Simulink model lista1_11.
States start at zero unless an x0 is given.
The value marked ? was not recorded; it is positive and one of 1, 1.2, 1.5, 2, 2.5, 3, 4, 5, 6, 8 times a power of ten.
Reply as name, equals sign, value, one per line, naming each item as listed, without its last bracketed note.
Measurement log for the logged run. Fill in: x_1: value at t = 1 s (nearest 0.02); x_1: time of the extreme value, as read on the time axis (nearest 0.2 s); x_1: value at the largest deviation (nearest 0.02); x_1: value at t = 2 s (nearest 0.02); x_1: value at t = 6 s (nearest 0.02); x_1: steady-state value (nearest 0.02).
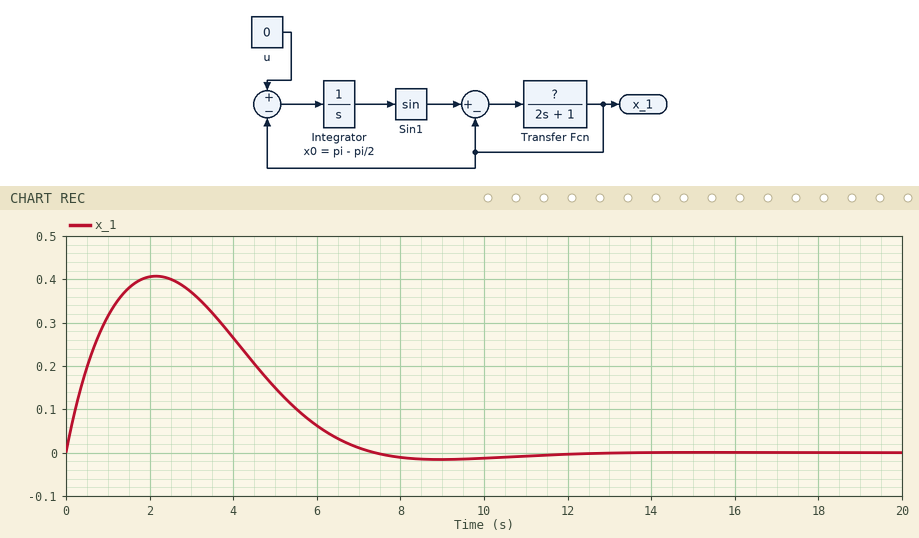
x_1: value at t = 1 s = 0.32
x_1: time of the extreme value, as read on the time axis = 2.2 s
x_1: value at the largest deviation = 0.40
x_1: value at t = 2 s = 0.40
x_1: value at t = 6 s = 0.06
x_1: steady-state value = 0.00
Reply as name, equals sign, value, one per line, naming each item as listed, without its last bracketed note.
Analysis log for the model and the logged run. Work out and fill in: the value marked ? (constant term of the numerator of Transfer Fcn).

the value marked ? = 1
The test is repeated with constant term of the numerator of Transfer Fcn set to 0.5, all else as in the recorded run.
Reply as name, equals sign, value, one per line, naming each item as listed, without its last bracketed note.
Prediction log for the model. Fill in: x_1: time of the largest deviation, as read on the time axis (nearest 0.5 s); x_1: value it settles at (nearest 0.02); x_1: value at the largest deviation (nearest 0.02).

x_1: time of the largest deviation, as read on the time axis = 3.0 s
x_1: value it settles at = 0.00
x_1: value at the largest deviation = 0.28
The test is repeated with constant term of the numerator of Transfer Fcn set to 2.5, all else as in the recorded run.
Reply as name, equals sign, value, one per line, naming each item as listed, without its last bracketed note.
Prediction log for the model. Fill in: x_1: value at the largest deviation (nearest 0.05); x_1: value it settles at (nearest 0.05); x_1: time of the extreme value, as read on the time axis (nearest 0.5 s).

x_1: value at the largest deviation = 0.60
x_1: value it settles at = 0.00
x_1: time of the extreme value, as read on the time axis = 1.5 s
